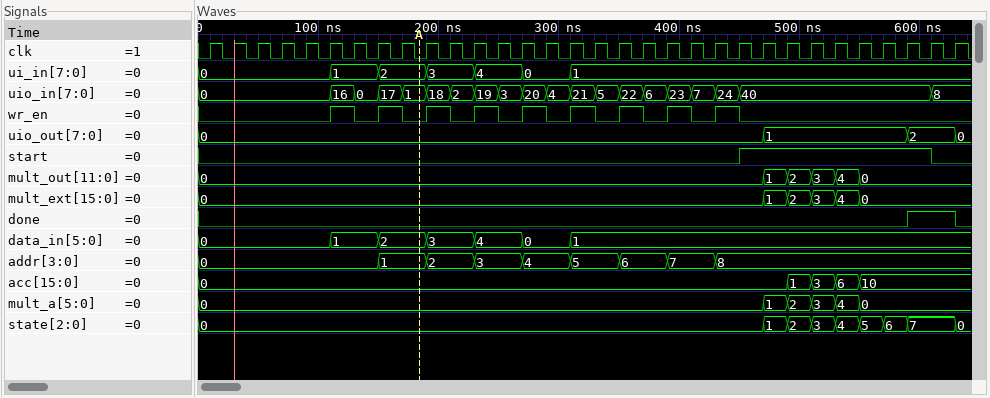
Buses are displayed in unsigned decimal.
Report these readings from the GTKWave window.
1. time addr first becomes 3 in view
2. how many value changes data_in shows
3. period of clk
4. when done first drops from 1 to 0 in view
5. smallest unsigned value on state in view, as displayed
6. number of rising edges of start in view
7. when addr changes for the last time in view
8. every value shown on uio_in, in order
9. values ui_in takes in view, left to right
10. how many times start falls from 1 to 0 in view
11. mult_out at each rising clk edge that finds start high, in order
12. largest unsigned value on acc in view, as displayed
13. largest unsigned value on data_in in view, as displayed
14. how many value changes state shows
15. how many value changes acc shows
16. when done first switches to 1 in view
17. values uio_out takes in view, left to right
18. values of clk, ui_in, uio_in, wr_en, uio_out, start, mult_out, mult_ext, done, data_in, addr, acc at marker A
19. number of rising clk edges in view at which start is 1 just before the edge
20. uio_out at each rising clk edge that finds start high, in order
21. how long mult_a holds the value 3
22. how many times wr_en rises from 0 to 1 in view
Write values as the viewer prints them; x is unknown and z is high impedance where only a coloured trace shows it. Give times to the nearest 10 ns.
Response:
230 ns
6
20 ns
630 ns
0
1
430 ns
0, 16, 0, 17, 1, 18, 2, 19, 3, 20, 4, 21, 5, 22, 6, 23, 7, 24, 40, 8
0, 1, 2, 3, 4, 0, 1
1
0, 1, 2, 3, 4, 0, 0, 0
10
4
8
4
590 ns
0, 1, 2, 0
clk=0, ui_in=2, uio_in=1, wr_en=0, uio_out=0, start=0, mult_out=0, mult_ext=0, done=0, data_in=2, addr=1, acc=0
8
0, 1, 1, 1, 1, 1, 1, 2
20 ns
9
